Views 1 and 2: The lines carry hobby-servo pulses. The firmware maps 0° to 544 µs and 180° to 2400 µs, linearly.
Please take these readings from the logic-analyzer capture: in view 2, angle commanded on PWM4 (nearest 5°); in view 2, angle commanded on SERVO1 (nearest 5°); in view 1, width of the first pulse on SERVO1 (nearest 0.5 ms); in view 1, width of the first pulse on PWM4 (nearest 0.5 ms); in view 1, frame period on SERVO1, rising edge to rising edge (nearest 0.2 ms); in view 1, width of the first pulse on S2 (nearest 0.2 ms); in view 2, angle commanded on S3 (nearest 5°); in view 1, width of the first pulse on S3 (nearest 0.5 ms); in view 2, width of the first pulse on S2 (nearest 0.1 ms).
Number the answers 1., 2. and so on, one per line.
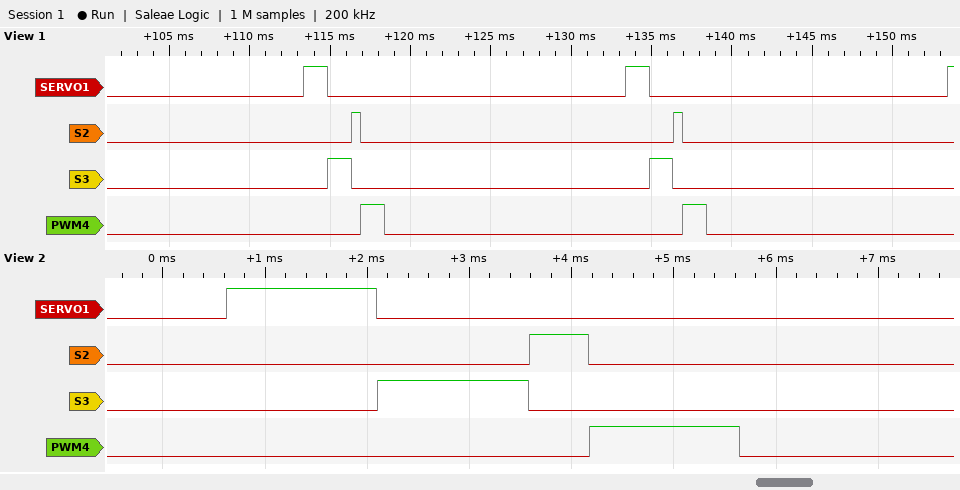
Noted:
1. 90°
2. 90°
3. 1.5 ms
4. 1.5 ms
5. 20.0 ms
6. 0.6 ms
7. 90°
8. 1.5 ms
9. 0.6 ms
